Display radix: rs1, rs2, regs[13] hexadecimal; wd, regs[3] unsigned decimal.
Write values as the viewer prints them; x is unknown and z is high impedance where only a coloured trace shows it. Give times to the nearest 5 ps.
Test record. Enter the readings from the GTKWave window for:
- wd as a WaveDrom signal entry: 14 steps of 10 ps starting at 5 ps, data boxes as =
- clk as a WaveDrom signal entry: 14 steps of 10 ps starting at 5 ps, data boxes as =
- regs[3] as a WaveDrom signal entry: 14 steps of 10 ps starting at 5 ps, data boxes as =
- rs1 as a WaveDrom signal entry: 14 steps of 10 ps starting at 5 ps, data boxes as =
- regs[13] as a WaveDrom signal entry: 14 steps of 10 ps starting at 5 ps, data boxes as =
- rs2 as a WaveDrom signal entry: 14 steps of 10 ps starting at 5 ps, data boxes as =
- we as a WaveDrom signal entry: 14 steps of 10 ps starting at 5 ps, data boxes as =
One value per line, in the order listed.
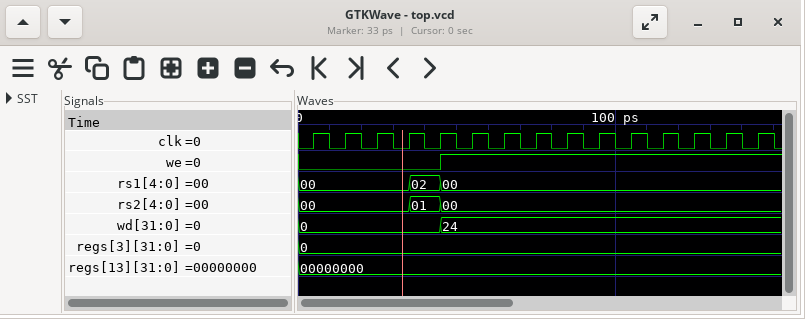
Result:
{name: 'wd', wave: '=...=.........', data: '0 24'}
{name: 'clk', wave: 'p.............'}
{name: 'regs[3]', wave: '=.............', data: '0'}
{name: 'rs1', wave: '=..==.........', data: '00 02 00'}
{name: 'regs[13]', wave: '=.............', data: '00000000'}
{name: 'rs2', wave: '=..==.........', data: '00 01 00'}
{name: 'we', wave: '0...1.........'}
